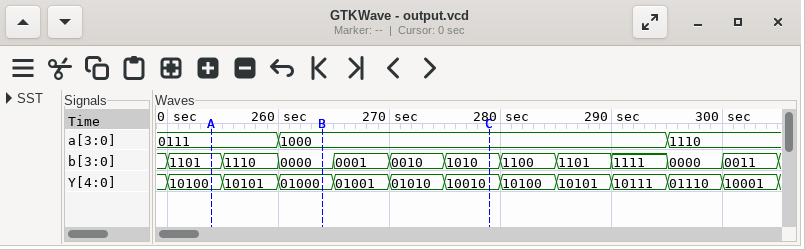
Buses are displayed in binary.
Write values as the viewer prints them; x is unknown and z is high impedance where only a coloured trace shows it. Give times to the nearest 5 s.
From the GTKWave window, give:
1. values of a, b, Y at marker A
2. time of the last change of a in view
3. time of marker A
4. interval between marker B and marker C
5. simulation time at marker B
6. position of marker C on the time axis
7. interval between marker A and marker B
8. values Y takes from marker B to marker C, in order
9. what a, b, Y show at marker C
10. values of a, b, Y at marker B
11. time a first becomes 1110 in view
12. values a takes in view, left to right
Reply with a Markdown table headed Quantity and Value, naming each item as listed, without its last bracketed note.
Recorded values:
| Quantity | Value |
|---|---|
| values of a, b, Y at marker A | a=0111, b=1101, Y=10100 |
| time of the last change of a in view | 295 s |
| time of marker A | 255 s |
| interval between marker B and marker C | 15 s |
| simulation time at marker B | 265 s |
| position of marker C on the time axis | 280 s |
| interval between marker A and marker B | 10 s |
| values Y takes from marker B to marker C, in order | 01000, 01001, 01010, 10010 |
| what a, b, Y show at marker C | a=1000, b=1010, Y=10010 |
| values of a, b, Y at marker B | a=1000, b=0000, Y=01000 |
| time a first becomes 1110 in view | 295 s |
| values a takes in view, left to right | 0111, 1000, 1110 |
